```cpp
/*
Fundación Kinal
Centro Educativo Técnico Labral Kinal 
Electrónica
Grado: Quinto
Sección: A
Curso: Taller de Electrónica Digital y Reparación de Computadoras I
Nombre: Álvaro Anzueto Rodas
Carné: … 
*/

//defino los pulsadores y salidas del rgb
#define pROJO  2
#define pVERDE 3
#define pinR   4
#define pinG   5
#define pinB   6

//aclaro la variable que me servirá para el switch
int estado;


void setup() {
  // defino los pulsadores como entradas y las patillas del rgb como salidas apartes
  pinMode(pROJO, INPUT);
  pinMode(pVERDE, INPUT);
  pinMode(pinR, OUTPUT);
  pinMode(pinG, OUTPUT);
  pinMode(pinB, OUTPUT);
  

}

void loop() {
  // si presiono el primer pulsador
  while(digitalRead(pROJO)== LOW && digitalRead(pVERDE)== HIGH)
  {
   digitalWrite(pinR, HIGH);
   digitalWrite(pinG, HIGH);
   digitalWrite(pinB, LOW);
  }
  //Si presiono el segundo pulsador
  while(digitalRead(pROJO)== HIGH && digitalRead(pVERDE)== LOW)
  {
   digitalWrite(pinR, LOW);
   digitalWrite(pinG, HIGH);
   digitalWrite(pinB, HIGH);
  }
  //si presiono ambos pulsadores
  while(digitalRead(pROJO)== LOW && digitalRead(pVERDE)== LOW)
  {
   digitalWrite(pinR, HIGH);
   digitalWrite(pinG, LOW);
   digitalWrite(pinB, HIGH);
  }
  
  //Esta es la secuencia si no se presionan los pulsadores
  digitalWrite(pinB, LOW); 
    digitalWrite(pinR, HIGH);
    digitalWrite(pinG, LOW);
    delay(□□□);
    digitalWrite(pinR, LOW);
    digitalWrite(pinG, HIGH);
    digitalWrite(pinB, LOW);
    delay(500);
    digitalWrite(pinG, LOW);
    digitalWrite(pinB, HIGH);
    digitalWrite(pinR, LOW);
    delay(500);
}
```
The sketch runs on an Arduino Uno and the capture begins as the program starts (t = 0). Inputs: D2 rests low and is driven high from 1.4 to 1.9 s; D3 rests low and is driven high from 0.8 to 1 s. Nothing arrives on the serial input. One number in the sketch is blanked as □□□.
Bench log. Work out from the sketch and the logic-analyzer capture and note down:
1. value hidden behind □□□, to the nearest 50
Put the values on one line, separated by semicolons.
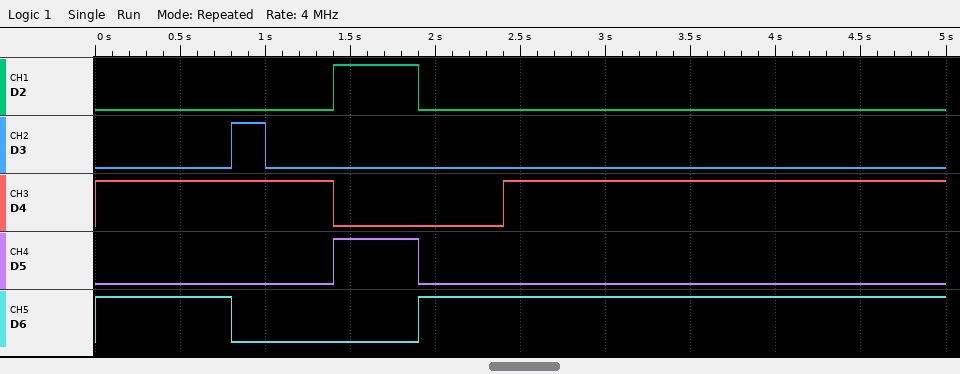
600
